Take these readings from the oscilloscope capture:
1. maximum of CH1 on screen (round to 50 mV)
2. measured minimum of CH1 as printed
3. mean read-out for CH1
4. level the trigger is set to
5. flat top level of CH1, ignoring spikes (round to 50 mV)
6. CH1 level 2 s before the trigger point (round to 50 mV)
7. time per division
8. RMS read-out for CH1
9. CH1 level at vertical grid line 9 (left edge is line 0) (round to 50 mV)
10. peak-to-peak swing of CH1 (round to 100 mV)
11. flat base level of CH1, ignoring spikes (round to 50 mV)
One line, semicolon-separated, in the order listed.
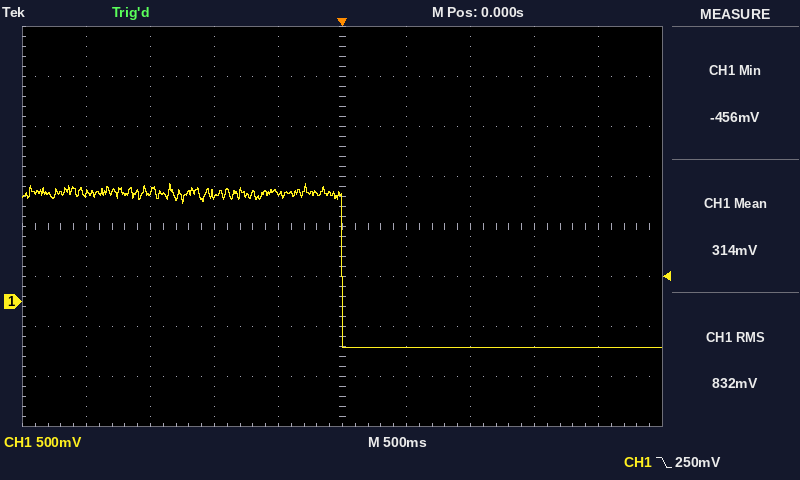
1.20 V; -456 mV; 314 mV; 250 mV; 1.10 V; 1.10 V; 500 ms; 832 mV; -450 mV; 1.60 V; -450 mV
